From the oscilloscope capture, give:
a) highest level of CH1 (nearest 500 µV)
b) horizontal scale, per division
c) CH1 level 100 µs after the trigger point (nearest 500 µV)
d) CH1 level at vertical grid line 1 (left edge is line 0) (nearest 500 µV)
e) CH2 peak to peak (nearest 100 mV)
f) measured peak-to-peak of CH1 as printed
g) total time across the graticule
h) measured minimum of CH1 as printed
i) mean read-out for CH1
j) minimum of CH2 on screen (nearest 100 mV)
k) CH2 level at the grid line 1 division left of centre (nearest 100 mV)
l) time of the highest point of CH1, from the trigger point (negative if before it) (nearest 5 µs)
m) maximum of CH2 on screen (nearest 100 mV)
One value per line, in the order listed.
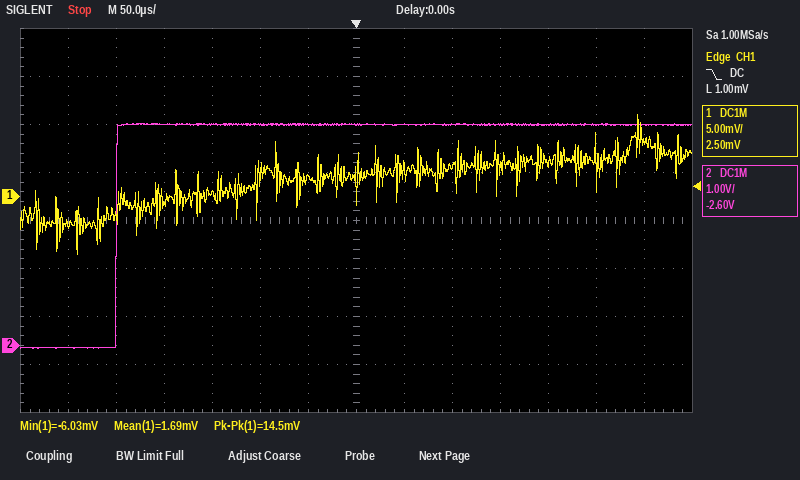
8.5 mV
50 µs
3.0 mV
-3.0 mV
4.7 V
14.5 mV
700 µs
-6.03 mV
1.69 mV
-100 mV
4.6 V
+295 µs
4.6 V
